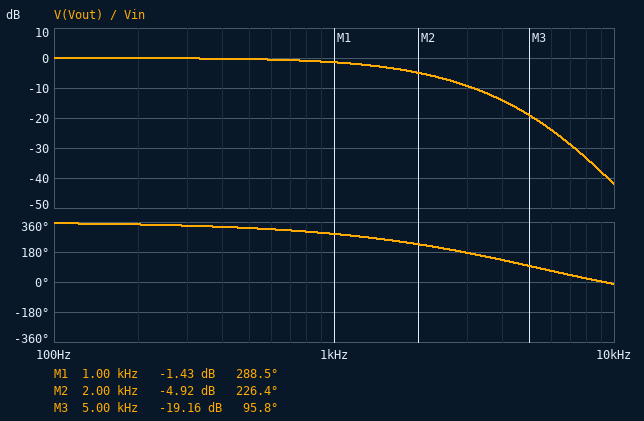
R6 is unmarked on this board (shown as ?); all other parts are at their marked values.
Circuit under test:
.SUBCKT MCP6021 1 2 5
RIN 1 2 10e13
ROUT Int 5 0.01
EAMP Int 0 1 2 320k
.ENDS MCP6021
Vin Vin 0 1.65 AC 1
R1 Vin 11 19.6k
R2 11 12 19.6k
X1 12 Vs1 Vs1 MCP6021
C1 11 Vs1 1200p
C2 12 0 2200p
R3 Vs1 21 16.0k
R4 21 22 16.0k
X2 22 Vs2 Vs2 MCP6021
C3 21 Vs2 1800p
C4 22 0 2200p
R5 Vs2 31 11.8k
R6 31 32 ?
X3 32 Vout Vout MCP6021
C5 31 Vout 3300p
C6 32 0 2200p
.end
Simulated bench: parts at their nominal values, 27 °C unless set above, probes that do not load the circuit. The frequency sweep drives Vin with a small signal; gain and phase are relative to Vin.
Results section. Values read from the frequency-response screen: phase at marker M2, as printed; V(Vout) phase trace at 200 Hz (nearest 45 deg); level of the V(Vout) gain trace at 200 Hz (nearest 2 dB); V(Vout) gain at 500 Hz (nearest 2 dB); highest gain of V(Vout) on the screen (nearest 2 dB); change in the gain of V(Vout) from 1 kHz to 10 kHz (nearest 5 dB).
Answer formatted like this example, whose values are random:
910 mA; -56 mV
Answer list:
226.4 deg; 360 deg; 0 dB; 0 dB; 0 dB; -40 dB
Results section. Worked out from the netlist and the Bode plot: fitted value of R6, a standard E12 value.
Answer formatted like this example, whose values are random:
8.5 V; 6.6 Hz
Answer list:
10 kΩ
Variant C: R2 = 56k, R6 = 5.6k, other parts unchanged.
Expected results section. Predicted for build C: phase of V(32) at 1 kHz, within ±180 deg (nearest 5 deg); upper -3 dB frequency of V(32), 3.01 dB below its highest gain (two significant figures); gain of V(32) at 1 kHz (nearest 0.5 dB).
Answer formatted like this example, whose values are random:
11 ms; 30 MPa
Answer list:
-90 deg; 940 Hz; -3.5 dB
